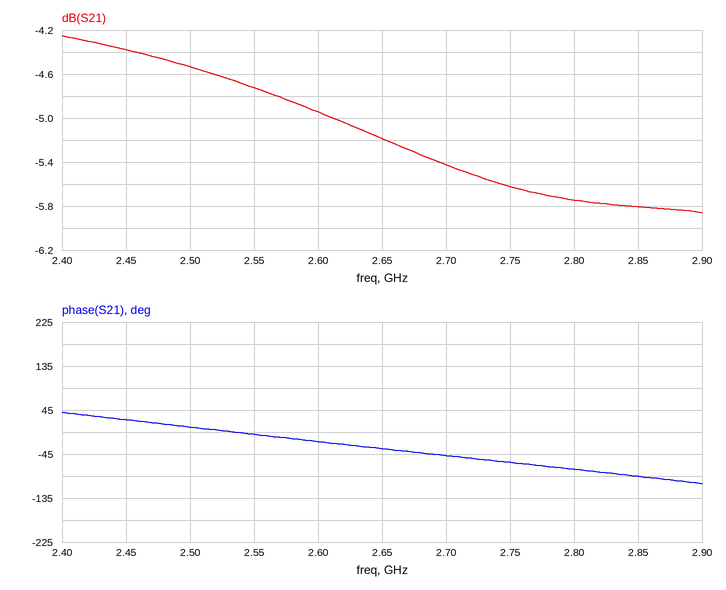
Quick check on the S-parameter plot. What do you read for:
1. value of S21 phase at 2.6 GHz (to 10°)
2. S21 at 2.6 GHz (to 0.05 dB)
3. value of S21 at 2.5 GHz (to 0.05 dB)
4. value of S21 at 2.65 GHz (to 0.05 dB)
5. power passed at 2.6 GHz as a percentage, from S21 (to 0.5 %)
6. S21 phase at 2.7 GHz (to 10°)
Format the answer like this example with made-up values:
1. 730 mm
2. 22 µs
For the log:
1. -20°
2. -4.95 dB
3. -4.55 dB
4. -5.20 dB
5. 32.0 %
6. -50°
